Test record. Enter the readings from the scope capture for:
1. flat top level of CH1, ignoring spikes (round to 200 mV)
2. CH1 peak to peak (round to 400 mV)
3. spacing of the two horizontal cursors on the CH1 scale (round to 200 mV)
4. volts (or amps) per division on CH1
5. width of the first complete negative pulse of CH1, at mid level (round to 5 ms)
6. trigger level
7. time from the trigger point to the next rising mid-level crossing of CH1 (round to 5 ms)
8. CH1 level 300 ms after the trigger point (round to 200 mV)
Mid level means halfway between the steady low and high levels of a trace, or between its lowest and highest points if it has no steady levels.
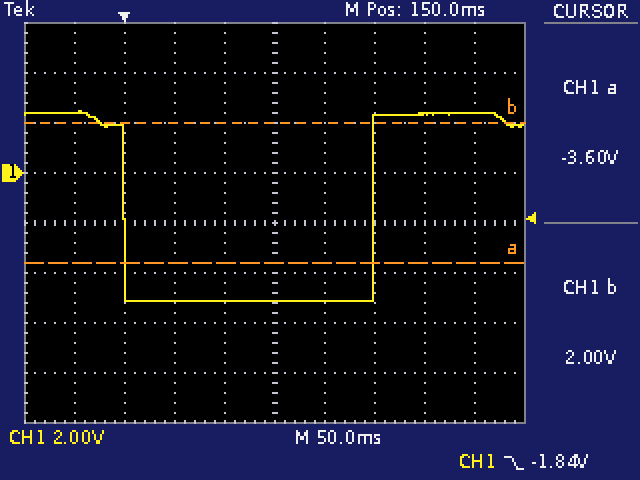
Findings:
2.4 V
7.6 V
5.6 V
2 V
250 ms
-1.84 V
250 ms
2.4 V
